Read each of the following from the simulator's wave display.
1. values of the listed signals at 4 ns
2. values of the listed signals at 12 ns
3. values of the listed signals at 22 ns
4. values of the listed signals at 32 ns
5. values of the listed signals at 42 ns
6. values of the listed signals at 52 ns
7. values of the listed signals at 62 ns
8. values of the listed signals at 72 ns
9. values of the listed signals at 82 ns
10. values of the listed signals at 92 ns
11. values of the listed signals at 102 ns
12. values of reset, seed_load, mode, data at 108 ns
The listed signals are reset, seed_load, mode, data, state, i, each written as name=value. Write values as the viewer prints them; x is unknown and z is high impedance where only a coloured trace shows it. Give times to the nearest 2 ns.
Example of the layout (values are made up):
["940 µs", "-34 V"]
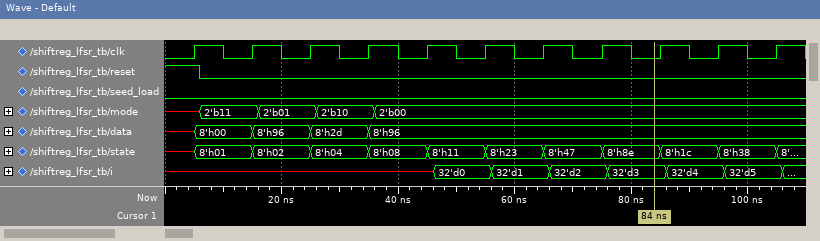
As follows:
["reset=1, seed_load=0, mode=x, data=x, state=x, i=x", "reset=0, seed_load=0, mode=2'b11, data=8'h00, state=8'h01, i=x", "reset=0, seed_load=0, mode=2'b01, data=8'h96, state=8'h02, i=x", "reset=0, seed_load=0, mode=2'b10, data=8'h2d, state=8'h04, i=x", "reset=0, seed_load=0, mode=2'b00, data=8'h96, state=8'h08, i=x", "reset=0, seed_load=0, mode=2'b00, data=8'h96, state=8'h11, i=32'd0", "reset=0, seed_load=0, mode=2'b00, data=8'h96, state=8'h23, i=32'd1", "reset=0, seed_load=0, mode=2'b00, data=8'h96, state=8'h47, i=32'd2", "reset=0, seed_load=0, mode=2'b00, data=8'h96, state=8'h8e, i=32'd3", "reset=0, seed_load=0, mode=2'b00, data=8'h96, state=8'h1c, i=32'd4", "reset=0, seed_load=0, mode=2'b00, data=8'h96, state=8'h38, i=32'd5", "reset=0, seed_load=0, mode=2'b00, data=8'h96"]
